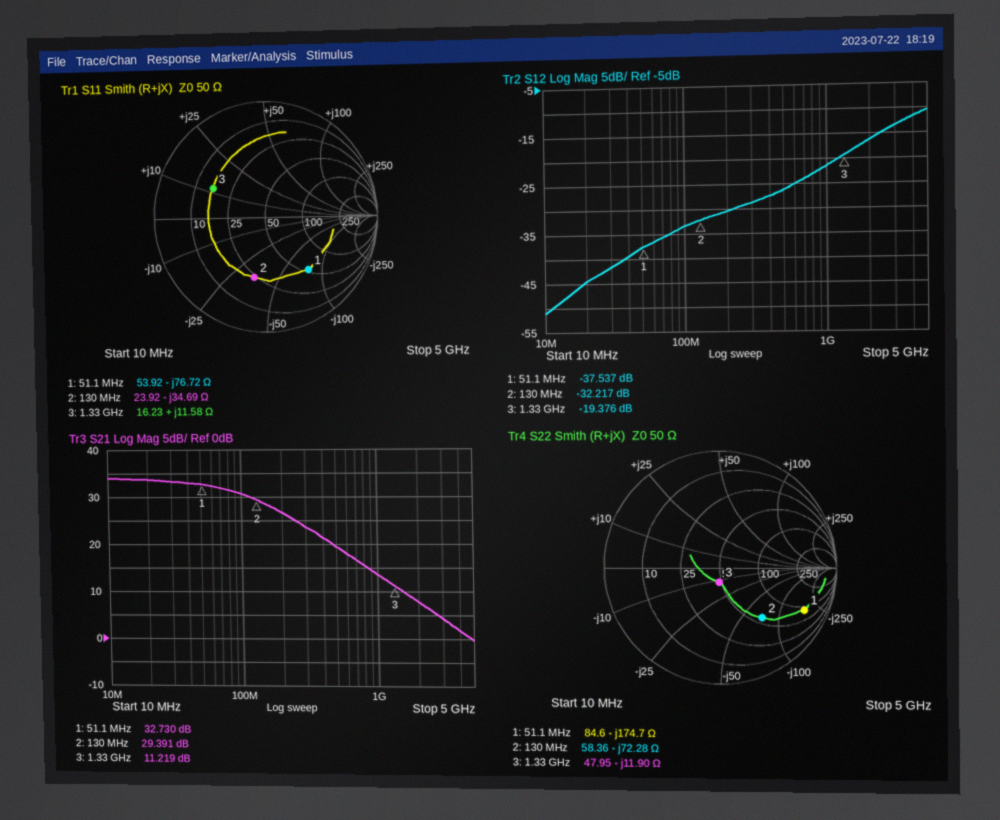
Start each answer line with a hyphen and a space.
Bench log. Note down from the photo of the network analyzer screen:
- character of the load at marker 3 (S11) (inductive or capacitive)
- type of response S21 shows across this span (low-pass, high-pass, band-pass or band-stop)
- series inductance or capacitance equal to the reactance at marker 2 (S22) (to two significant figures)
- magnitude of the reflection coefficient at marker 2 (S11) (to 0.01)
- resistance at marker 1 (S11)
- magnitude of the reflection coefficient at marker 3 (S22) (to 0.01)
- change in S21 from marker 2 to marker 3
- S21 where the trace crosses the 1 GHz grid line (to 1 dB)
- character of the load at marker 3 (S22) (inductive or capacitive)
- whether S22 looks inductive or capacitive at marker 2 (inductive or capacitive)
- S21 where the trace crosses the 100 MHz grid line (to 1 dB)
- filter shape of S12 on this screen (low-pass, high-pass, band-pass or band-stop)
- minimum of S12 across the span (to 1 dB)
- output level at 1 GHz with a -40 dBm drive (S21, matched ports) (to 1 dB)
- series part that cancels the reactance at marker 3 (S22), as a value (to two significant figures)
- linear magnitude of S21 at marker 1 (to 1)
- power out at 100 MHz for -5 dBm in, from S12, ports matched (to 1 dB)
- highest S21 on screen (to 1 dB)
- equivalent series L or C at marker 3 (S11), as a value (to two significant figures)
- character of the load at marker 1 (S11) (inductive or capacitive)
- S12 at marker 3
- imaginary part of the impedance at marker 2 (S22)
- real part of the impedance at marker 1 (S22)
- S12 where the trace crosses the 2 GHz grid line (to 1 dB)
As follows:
- inductive
- low-pass
- 17 pF
- 0.53
- 53.92 Ω
- 0.12
- -18.172 dB
- 14 dB
- capacitive
- capacitive
- 31 dB
- high-pass
- -51 dB
- -26 dBm
- 1.4 nH
- 43
- -38 dBm
- 34 dB
- 1.4 nH
- capacitive
- -19.376 dB
- -72.28 Ω
- 84.6 Ω
- -16 dB
